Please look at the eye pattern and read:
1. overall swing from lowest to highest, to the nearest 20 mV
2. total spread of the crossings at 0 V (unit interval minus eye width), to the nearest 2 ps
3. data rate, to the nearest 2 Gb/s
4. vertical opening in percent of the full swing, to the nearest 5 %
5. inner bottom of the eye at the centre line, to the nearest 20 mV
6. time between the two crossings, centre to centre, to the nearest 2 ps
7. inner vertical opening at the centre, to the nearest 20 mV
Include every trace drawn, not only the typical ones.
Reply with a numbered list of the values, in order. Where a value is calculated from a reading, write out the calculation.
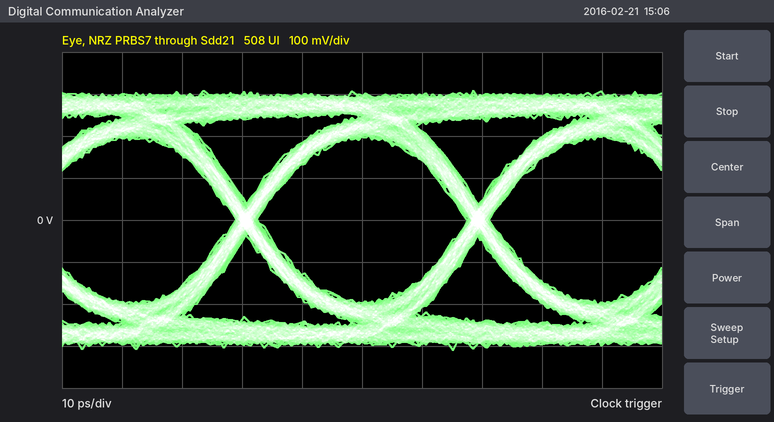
1. 620 mV
2. 4 ps
3. 26 Gb/s
4. 400 mV / 620 mV ≈ 65 %
5. -200 mV
6. 38 ps
7. 400 mV
